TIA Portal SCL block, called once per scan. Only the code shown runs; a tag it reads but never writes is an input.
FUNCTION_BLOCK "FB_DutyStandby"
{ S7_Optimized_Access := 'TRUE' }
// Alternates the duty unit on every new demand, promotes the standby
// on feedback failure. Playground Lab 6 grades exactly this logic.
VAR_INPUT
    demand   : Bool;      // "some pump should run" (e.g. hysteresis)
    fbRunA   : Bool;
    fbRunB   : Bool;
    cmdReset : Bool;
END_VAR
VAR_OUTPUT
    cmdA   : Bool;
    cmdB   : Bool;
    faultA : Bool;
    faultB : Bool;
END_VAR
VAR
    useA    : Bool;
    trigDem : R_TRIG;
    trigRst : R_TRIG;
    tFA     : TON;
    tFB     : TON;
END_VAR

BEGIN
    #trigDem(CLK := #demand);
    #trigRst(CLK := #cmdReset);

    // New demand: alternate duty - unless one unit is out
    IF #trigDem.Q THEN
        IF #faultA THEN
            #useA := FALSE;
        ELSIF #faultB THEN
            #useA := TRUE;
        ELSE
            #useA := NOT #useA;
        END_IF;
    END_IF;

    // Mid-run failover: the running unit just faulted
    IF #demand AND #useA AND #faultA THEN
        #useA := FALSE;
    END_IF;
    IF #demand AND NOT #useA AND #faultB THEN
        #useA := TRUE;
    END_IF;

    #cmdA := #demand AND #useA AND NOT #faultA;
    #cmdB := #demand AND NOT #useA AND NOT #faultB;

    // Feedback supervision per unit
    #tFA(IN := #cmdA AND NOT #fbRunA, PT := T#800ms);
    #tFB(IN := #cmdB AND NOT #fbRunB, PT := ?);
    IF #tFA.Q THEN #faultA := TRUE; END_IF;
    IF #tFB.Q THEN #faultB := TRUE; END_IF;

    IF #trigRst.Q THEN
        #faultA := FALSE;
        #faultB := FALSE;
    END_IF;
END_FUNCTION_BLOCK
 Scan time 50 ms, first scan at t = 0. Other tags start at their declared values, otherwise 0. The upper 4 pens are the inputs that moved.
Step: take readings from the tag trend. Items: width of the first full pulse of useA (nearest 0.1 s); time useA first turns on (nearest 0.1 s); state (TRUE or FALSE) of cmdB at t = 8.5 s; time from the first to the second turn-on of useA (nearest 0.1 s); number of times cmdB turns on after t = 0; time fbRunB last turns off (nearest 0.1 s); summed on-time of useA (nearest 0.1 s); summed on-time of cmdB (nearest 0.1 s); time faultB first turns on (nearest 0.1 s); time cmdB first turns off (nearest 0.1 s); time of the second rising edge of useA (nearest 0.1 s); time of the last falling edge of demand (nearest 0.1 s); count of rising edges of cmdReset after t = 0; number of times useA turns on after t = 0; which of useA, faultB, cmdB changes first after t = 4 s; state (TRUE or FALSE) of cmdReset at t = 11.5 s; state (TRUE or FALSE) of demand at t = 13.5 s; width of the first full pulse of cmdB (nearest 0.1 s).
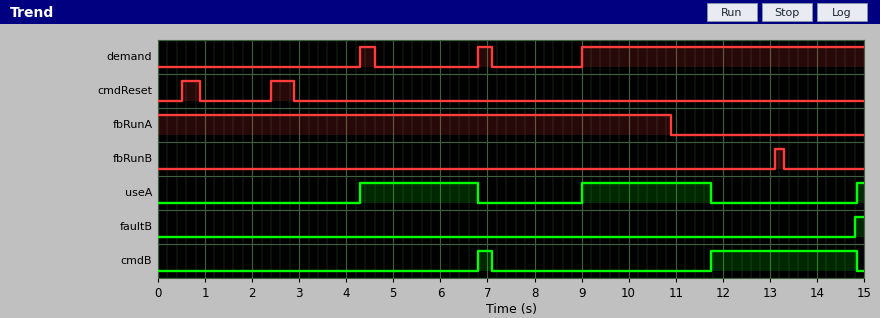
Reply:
2.5 s
4.3 s
FALSE
4.7 s
2
13.3 s
5.4 s
3.4 s
14.8 s
7.1 s
9.0 s
7.1 s
2
3
useA
FALSE
TRUE
0.3 s
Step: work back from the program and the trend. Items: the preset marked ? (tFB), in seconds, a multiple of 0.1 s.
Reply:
1.5 s
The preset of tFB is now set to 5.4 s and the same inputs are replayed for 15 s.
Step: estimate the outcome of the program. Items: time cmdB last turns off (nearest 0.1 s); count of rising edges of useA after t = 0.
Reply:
7.1 s
2
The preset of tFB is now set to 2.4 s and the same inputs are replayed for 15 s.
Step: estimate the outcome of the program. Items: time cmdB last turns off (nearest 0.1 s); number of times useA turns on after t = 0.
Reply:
7.1 s
2
